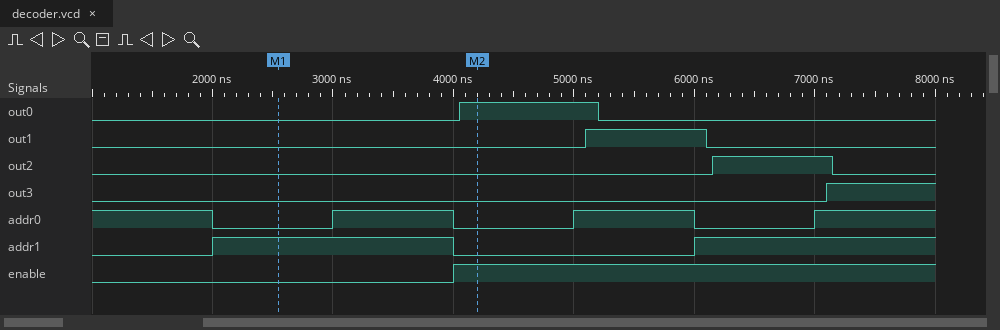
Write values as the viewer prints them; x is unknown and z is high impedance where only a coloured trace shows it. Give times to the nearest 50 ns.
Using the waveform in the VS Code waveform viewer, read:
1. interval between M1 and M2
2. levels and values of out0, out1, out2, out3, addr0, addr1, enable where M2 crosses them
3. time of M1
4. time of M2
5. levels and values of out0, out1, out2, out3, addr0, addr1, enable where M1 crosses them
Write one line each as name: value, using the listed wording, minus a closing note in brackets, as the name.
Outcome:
interval between M1 and M2: 1650 ns
levels and values of out0, out1, out2, out3, addr0, addr1, enable where M2 crosses them: out0=1, out1=0, out2=0, out3=0, addr0=0, addr1=0, enable=1
time of M1: 2550 ns
time of M2: 4200 ns
levels and values of out0, out1, out2, out3, addr0, addr1, enable where M1 crosses them: out0=0, out1=0, out2=0, out3=0, addr0=0, addr1=1, enable=0
